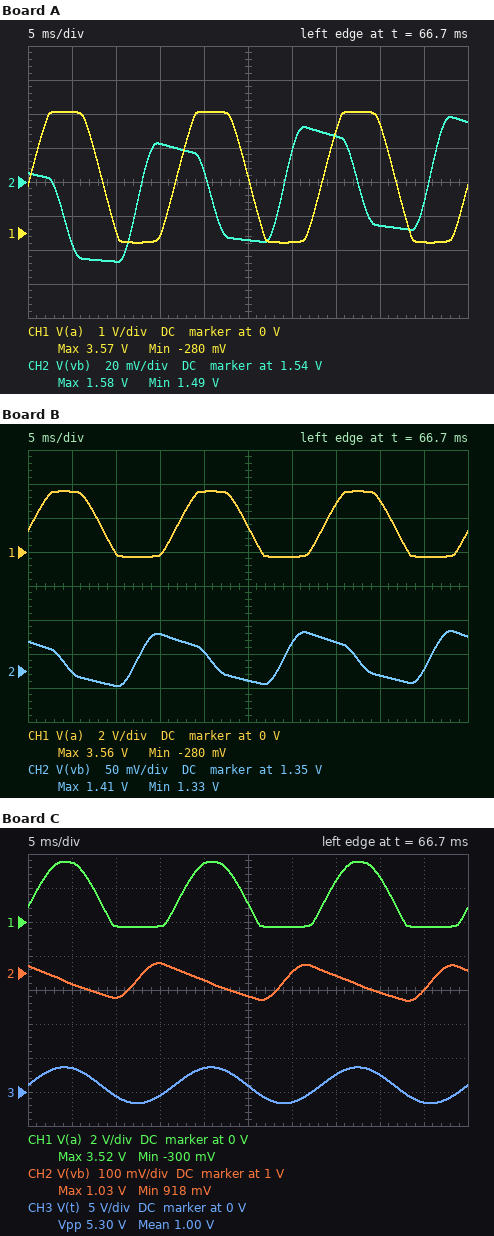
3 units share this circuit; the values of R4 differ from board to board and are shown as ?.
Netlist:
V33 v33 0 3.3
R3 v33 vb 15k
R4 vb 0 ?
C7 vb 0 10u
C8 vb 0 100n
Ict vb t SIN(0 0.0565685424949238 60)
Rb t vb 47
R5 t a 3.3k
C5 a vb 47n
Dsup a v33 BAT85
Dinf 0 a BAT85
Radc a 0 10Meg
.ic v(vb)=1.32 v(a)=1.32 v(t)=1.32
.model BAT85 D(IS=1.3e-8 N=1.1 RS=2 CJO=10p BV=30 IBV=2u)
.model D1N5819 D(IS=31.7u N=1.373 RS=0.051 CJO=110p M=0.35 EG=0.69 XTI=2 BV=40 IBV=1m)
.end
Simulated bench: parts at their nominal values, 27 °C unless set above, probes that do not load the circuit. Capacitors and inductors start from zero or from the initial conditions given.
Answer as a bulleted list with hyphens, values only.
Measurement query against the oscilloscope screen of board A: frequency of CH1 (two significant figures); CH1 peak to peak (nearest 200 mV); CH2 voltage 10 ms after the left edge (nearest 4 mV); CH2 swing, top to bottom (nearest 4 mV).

- 60 Hz
- 3.8 V
- 1.492 V
- 84 mV
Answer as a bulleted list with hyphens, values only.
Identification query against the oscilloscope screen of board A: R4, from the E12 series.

- 12 kΩ
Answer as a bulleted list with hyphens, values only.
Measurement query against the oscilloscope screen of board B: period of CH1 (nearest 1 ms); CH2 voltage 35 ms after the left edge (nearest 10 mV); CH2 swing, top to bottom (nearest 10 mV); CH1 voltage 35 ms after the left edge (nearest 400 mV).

- 17 ms
- 1.39 V
- 80 mV
- 2.8 V
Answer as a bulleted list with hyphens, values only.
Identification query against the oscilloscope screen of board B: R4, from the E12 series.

- 8.2 kΩ
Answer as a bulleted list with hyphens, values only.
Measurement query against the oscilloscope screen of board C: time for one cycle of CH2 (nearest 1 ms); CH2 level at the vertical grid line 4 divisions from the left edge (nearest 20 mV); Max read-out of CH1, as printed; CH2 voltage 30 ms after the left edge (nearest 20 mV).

- 17 ms
- 980 mV
- 3.52 V
- 1.00 V
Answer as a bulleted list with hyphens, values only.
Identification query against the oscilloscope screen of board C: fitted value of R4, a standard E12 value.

- 3.9 kΩ
